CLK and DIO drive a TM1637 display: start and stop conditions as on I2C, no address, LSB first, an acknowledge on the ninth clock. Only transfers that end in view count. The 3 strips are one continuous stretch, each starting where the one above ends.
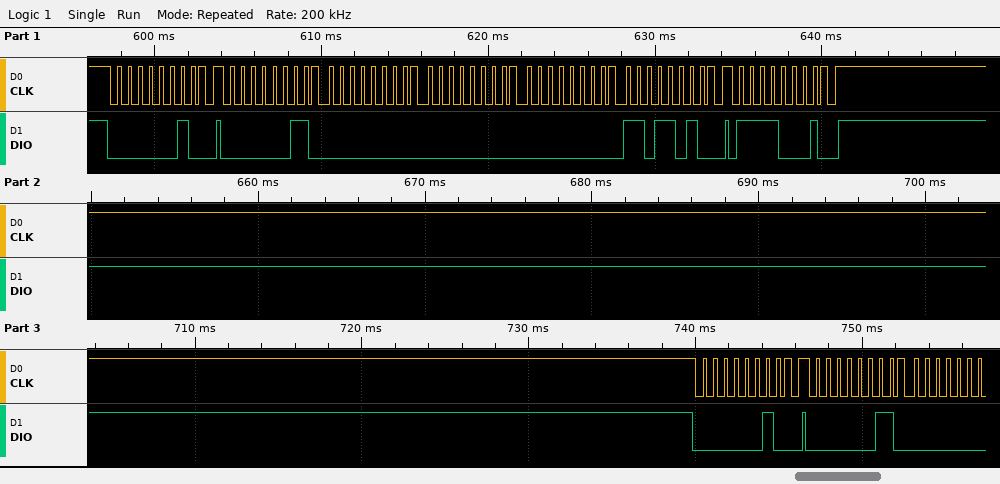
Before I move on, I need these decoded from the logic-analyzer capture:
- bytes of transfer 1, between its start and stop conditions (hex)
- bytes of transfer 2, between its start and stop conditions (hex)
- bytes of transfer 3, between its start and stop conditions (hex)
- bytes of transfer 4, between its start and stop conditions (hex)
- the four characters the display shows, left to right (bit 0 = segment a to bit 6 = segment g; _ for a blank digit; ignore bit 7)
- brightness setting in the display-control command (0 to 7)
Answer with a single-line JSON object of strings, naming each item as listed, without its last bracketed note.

{"bytes of transfer 1, between its start and stop conditions": "40", "bytes of transfer 2, between its start and stop conditions": "C0 00 00 00 5B", "bytes of transfer 3, between its start and stop conditions": "8F", "bytes of transfer 4, between its start and stop conditions": "40", "the four characters the display shows, left to right": "___2", "brightness setting in the display-control command": "7"}
